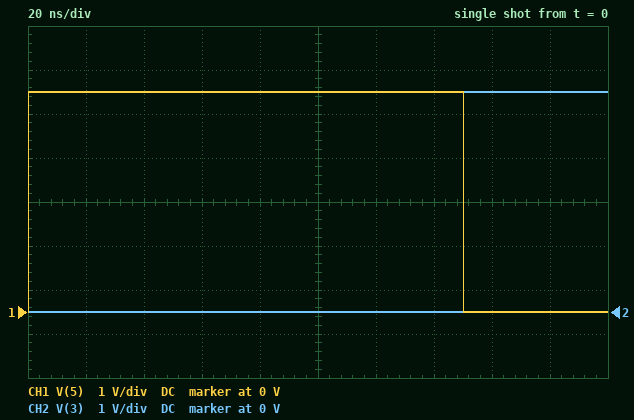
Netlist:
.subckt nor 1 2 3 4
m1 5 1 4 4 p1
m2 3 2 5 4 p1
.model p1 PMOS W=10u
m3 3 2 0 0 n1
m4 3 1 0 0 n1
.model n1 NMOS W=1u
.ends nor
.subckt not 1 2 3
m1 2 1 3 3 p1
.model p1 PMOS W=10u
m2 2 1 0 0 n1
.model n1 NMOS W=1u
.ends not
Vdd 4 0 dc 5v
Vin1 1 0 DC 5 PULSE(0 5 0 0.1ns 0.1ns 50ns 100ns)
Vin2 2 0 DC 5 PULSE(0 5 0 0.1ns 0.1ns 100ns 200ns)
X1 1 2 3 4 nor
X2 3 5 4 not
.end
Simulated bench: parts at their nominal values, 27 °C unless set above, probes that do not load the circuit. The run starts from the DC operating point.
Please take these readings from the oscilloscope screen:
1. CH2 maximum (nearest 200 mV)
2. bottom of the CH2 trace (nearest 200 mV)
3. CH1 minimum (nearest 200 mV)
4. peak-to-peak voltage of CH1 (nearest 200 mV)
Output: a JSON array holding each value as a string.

["5.0 V", "0 V", "0 V", "5.0 V"]
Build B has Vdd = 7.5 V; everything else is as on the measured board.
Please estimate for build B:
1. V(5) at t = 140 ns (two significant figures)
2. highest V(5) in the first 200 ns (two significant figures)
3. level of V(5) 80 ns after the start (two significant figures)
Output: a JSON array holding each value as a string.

["430 mV", "7.5 V", "480 mV"]
